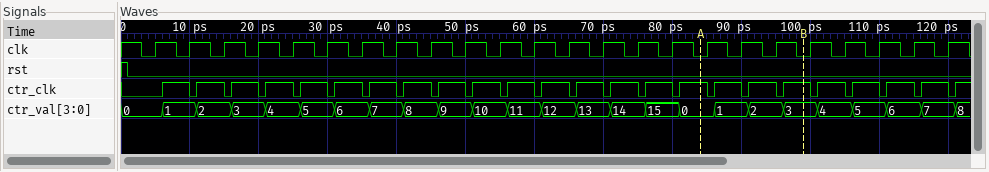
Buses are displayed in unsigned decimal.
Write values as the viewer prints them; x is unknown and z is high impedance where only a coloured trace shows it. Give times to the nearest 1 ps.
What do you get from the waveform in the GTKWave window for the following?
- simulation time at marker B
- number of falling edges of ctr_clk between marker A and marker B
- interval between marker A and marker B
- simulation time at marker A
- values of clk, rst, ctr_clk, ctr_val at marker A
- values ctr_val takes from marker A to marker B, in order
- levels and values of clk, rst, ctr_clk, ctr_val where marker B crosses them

99 ps
3
15 ps
84 ps
clk=0, rst=0, ctr_clk=1, ctr_val=0
0, 1, 2, 3
clk=0, rst=0, ctr_clk=1, ctr_val=3
